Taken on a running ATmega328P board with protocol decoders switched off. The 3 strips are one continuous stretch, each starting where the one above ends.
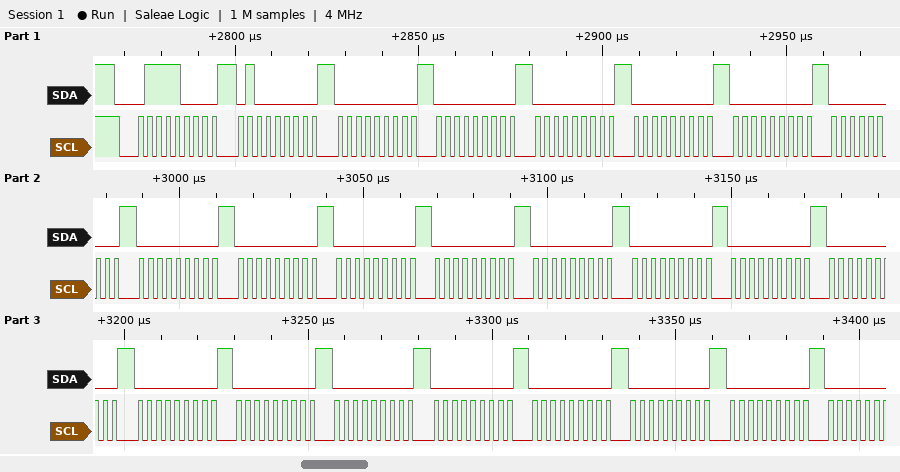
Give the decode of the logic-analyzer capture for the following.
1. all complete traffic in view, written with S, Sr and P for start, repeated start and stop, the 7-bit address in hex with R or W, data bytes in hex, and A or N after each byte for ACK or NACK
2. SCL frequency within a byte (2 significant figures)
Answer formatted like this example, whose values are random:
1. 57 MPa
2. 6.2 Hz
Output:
1. S 3CW A 40 A 00 A 00 A 00 A 00 A 00 A 00 A 00 A 00 A 00 A 00 A 00 A 00 A 00 A 00 A 00 A 00 A 00 A 00 A 00 A 00 A 00 A
2. 400 kHz
